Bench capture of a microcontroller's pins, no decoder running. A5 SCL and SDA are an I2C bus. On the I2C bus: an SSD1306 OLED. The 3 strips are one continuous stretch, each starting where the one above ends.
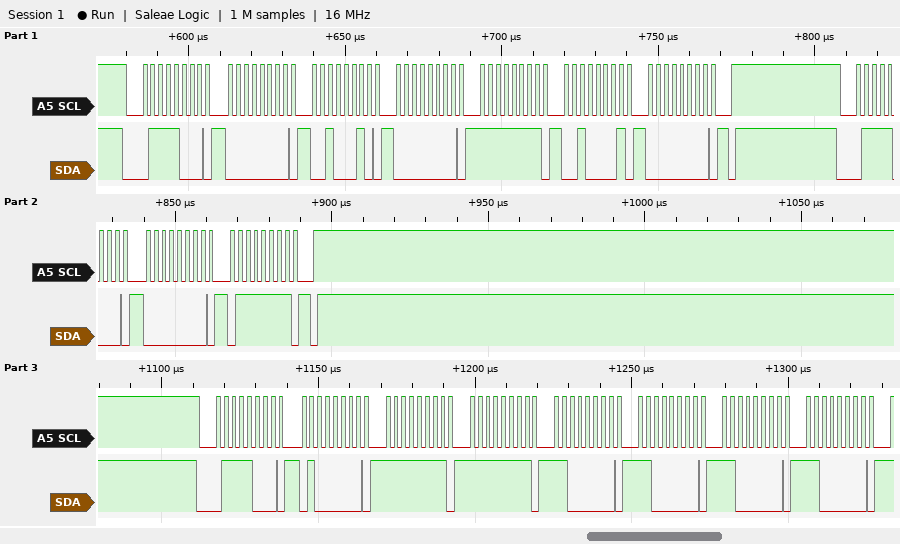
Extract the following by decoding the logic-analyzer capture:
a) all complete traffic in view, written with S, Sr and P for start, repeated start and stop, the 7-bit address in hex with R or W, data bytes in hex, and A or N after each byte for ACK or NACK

S 3CW A 00 A 22 A 00 A FF A 21 A 00 A P S 3CW A 00 A 7F A P S 3CW A 40 A FF A FF A C0 A C0 A C0 A C0 A
